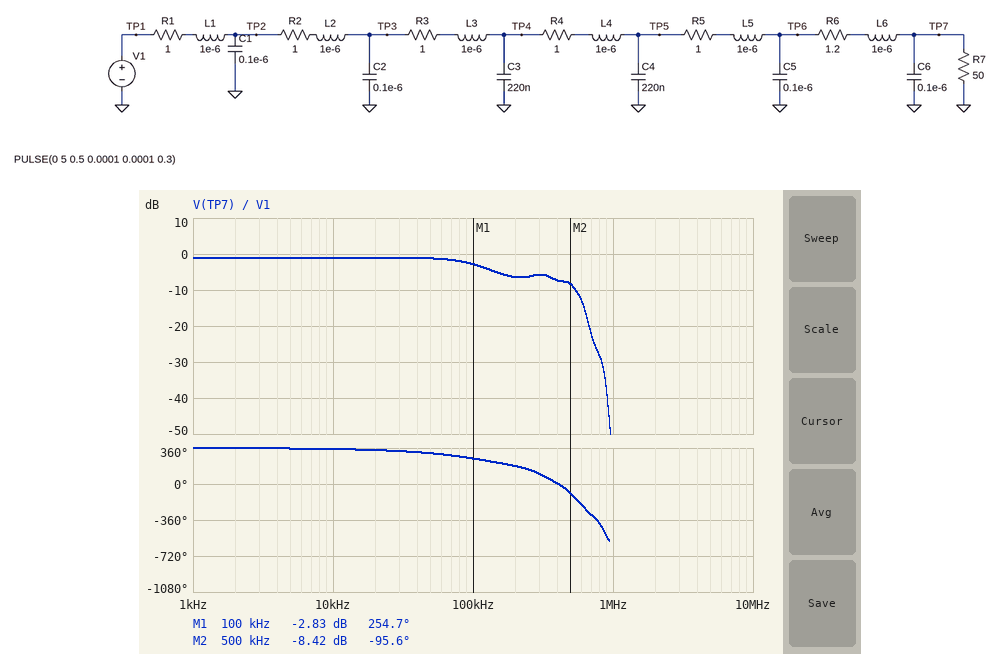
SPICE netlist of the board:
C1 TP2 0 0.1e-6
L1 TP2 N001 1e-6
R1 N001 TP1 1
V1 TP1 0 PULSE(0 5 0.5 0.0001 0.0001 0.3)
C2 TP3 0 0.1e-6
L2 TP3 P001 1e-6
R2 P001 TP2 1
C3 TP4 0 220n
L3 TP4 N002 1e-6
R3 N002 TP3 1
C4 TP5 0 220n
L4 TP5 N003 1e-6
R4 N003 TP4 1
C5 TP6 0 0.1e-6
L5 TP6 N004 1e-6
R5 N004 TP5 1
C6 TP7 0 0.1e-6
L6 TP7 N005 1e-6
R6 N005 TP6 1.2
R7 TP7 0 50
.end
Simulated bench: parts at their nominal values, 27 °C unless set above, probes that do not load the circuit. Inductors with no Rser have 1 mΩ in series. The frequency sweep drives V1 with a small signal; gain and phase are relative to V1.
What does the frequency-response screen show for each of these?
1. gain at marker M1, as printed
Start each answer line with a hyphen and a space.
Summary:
- -2.83 dB
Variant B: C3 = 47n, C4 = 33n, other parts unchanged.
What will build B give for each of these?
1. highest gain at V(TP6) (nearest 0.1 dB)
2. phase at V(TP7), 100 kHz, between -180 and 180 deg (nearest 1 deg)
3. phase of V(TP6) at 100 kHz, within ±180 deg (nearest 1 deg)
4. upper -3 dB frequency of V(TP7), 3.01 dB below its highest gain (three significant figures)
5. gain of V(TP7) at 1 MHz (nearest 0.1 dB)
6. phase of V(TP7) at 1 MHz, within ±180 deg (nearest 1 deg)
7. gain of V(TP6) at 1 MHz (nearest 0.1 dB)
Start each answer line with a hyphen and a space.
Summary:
- 0 dB
- -71 deg
- -66 deg
- 212 kHz
- -26.2 dB
- -27 deg
- -16.5 dB
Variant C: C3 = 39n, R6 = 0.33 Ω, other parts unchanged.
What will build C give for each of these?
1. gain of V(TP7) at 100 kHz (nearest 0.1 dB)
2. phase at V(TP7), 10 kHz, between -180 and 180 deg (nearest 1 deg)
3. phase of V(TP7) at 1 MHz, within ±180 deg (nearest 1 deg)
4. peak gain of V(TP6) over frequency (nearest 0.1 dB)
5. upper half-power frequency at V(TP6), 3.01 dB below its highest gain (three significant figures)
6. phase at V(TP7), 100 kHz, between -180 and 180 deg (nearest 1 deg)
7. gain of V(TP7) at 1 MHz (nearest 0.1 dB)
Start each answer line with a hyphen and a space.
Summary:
- -1.5 dB
- -8 deg
- -122 deg
- -0.7 dB
- 138 kHz
- -90 deg
- -42.8 dB
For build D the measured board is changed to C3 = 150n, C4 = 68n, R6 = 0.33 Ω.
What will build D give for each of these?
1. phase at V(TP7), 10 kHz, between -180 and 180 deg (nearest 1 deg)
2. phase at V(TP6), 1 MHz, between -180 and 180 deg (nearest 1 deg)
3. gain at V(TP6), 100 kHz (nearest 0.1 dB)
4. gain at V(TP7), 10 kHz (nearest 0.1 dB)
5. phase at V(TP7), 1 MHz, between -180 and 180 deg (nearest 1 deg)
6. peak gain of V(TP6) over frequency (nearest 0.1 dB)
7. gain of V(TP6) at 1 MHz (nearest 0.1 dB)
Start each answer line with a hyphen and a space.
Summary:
- -7 deg
- 5 deg
- -0.7 dB
- -0.9 dB
- -169 deg
- -0.4 dB
- -23.5 dB
